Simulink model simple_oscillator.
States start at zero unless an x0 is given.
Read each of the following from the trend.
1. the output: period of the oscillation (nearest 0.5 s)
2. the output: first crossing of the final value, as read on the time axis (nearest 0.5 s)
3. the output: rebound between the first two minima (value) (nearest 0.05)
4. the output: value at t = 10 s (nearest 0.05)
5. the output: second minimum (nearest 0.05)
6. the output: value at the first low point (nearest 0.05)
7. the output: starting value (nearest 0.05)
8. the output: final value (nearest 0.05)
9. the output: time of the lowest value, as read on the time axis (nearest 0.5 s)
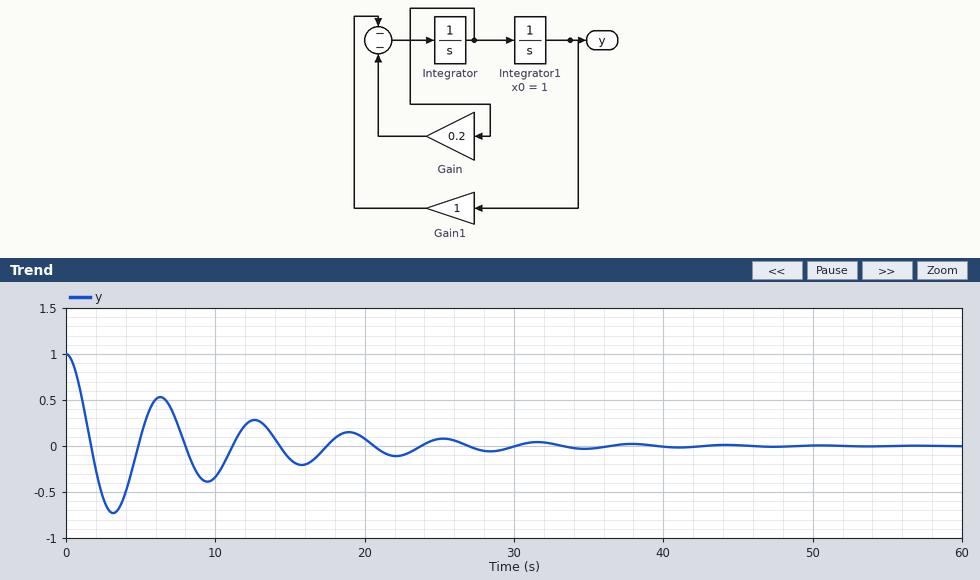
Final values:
6.5 s
1.5 s
0.55
-0.35
-0.40
-0.75
1.00
0.00
3.0 s
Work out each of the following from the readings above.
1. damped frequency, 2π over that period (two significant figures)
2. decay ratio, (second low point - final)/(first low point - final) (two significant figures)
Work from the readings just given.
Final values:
0.97 rad/s
0.53
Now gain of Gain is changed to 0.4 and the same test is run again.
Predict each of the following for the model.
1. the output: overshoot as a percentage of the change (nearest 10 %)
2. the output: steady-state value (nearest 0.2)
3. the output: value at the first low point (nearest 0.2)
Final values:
50 %
0.0
-0.6
